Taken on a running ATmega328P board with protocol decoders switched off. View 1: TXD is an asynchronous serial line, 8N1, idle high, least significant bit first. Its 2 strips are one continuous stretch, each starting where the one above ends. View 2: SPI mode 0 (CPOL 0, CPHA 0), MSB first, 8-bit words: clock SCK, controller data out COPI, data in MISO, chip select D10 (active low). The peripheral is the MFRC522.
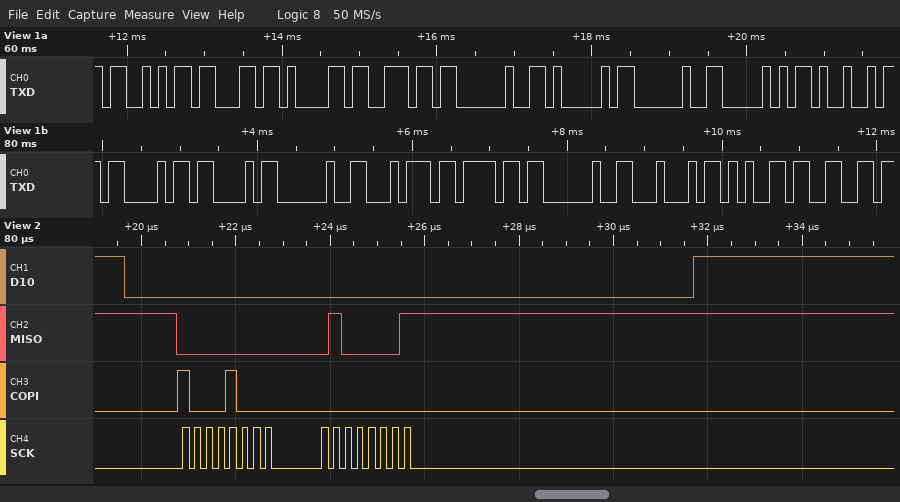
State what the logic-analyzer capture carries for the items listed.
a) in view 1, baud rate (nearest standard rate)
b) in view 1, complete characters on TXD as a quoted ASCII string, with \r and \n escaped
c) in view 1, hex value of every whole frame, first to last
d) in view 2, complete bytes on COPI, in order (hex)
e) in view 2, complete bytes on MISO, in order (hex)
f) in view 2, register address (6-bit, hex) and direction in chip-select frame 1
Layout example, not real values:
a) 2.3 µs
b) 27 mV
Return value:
a) 9600 baud
b) "Scan A PICC to Def"
c) 0x53 0x63 0x61 0x6E 0x20 0x41 0x20 0x50 0x49 0x43 0x43 0x20 0x74 0x6F 0x20 0x44 0x65 0x66
d) 88 00
e) 00 41
f) 0x04 read
